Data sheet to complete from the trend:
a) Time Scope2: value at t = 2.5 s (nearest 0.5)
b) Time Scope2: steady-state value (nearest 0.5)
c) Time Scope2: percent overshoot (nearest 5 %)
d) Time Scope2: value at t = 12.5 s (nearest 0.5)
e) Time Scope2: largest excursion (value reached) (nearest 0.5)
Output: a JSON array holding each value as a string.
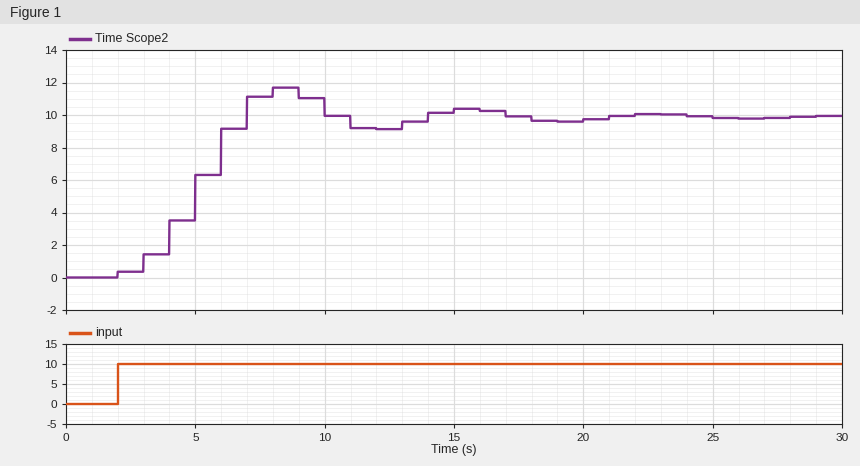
["0.5", "10.0", "20 %", "9.0", "11.5"]
